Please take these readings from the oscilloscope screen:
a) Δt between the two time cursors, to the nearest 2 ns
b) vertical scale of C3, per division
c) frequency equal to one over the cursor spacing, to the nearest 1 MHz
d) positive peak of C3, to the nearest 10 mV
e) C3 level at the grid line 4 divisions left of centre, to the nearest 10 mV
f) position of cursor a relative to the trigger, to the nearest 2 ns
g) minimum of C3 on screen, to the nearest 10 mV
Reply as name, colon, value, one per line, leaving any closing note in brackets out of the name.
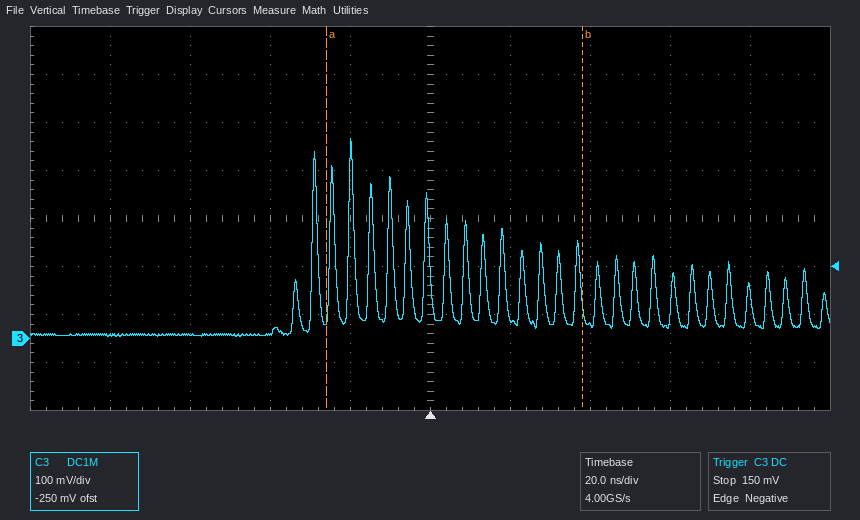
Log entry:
Δt between the two time cursors, to the nearest 2 ns: 64 ns
vertical scale of C3, per division: 100 mV
frequency equal to one over the cursor spacing, to the nearest 1 MHz: 16 MHz
positive peak of C3, to the nearest 10 mV: 420 mV
C3 level at the grid line 4 divisions left of centre, to the nearest 10 mV: 10 mV
position of cursor a relative to the trigger, to the nearest 2 ns: -26 ns
minimum of C3 on screen, to the nearest 10 mV: 0 mV
